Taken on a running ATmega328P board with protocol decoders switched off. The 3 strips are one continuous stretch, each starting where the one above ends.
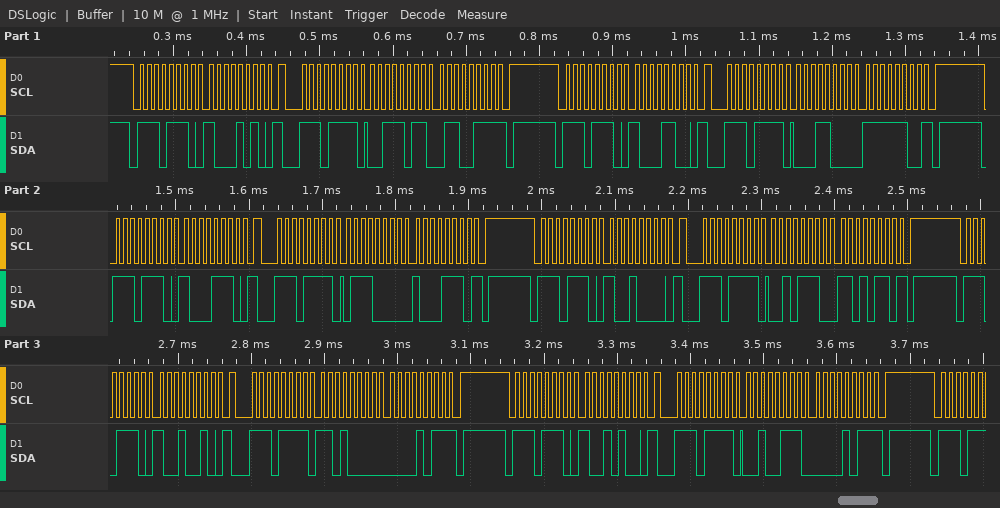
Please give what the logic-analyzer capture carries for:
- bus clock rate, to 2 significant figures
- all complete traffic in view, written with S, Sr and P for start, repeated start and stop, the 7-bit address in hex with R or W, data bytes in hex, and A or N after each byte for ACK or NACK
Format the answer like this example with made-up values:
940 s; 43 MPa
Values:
100 kHz; S 77W A 8A A Sr 77R A 3B A 67 N P S 77W A 8C A Sr 77R A 18 A FC N P S 77W A 8E A Sr 77R A 70 A 8E N P S 77W A 90 A Sr 77R A 2E A D6 N P S 77W A 92 A Sr 77R A D0 A 0B N P S 77W A 94 A Sr 77R A 27 A 0B N P
